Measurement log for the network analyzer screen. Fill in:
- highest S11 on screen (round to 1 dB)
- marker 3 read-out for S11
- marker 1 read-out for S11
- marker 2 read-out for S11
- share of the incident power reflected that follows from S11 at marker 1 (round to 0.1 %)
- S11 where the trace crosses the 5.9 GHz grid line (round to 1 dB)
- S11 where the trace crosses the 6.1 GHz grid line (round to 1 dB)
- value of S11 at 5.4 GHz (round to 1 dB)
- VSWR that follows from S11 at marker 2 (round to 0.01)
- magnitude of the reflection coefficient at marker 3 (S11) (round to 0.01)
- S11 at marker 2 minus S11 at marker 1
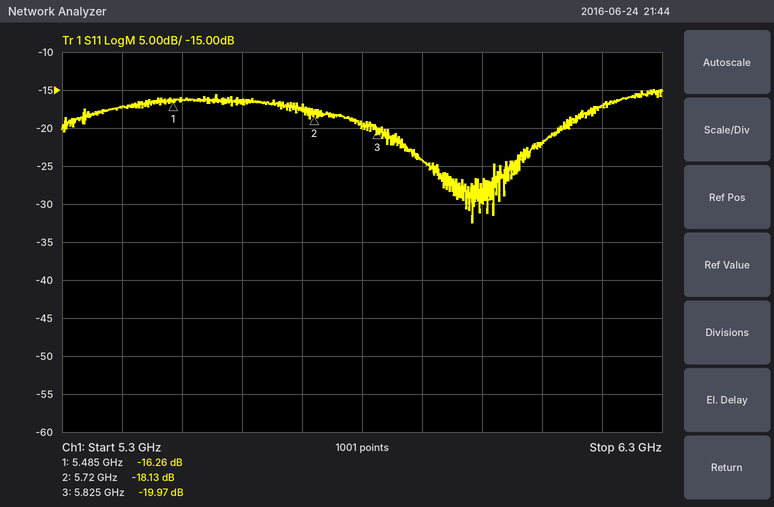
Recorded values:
-15 dB
-19.97 dB
-16.26 dB
-18.13 dB
2.4 %
-24 dB
-22 dB
-17 dB
1.28
0.10
-1.87 dB
